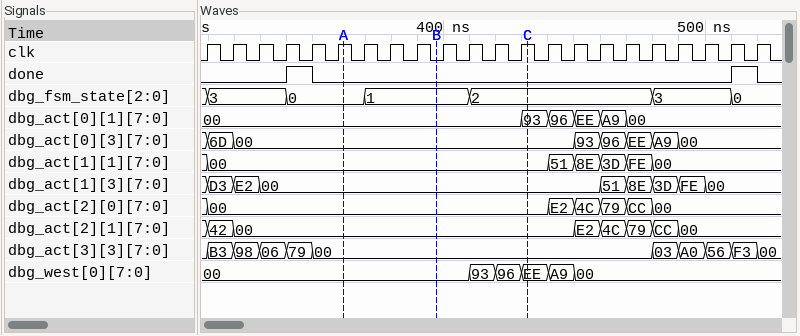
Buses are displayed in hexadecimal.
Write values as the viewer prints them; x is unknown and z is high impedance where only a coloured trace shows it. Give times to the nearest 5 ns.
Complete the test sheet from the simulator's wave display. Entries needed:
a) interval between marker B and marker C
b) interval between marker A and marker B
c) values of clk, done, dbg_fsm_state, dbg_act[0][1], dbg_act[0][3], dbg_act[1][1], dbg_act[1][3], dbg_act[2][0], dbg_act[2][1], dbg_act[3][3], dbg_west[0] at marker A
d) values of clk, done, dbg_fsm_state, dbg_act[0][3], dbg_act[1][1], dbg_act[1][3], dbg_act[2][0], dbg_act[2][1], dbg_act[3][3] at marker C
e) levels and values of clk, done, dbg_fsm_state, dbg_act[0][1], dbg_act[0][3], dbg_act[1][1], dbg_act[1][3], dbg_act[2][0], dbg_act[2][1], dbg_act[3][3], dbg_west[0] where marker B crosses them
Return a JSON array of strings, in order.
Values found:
["35 ns", "35 ns", "clk=1, done=0, dbg_fsm_state=0, dbg_act[0][1]=00, dbg_act[0][3]=00, dbg_act[1][1]=00, dbg_act[1][3]=00, dbg_act[2][0]=00, dbg_act[2][1]=00, dbg_act[3][3]=00, dbg_west[0]=00", "clk=1, done=0, dbg_fsm_state=2, dbg_act[0][3]=00, dbg_act[1][1]=00, dbg_act[1][3]=00, dbg_act[2][0]=00, dbg_act[2][1]=00, dbg_act[3][3]=00", "clk=0, done=0, dbg_fsm_state=1, dbg_act[0][1]=00, dbg_act[0][3]=00, dbg_act[1][1]=00, dbg_act[1][3]=00, dbg_act[2][0]=00, dbg_act[2][1]=00, dbg_act[3][3]=00, dbg_west[0]=00"]
